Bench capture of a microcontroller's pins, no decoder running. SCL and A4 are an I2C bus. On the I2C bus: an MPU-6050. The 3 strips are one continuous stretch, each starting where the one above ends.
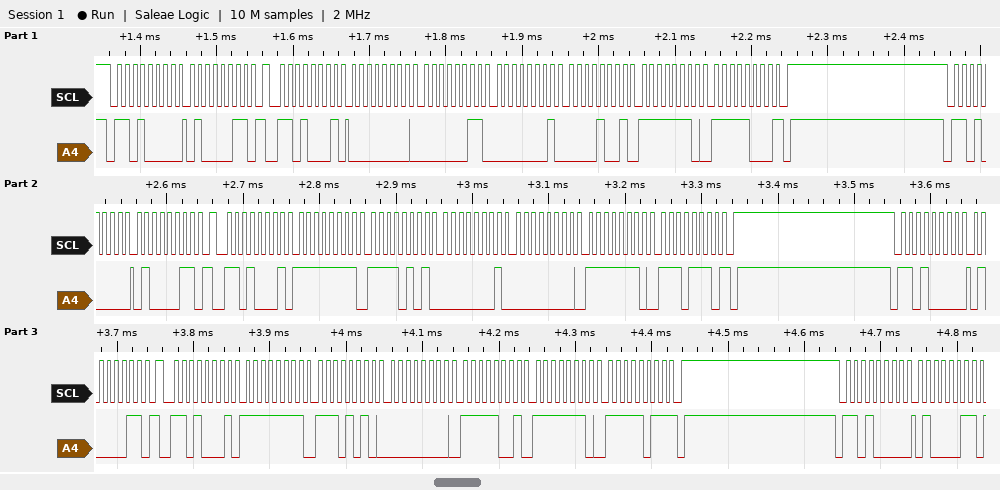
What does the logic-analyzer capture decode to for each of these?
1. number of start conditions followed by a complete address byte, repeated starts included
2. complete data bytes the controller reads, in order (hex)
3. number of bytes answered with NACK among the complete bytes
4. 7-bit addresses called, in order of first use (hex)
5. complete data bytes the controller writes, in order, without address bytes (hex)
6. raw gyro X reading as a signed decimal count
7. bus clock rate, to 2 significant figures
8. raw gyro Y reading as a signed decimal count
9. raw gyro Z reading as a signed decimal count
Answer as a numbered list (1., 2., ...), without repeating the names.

1. 7
2. 00 03 01 09 FE F8 FF F5 01 00 FE EE FF EA 00 F9 FE FB
3. 3
4. 0x68
5. 43 43 43 43
6. 3
7. 100 kHz
8. 265
9. -264
